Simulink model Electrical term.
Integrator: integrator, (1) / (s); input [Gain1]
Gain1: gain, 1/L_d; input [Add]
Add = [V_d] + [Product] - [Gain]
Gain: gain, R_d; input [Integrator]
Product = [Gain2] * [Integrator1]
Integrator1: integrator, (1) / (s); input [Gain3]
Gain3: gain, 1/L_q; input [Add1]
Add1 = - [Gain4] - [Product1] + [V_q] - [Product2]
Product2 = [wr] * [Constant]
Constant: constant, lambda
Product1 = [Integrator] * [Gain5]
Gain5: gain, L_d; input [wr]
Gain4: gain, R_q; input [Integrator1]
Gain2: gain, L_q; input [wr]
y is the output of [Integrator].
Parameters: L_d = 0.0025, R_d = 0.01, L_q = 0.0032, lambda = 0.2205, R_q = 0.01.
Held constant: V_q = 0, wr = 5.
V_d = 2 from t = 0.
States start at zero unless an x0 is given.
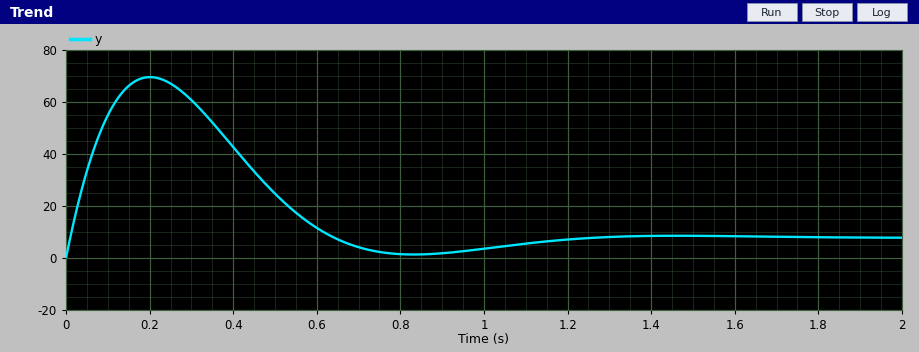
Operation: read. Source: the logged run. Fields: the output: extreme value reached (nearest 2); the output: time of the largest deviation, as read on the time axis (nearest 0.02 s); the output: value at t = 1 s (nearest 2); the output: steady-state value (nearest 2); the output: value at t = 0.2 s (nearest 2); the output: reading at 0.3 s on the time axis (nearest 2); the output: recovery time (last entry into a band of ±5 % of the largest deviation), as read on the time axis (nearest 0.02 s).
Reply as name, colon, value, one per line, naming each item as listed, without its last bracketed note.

the output: extreme value reached: 70
the output: time of the largest deviation, as read on the time axis: 0.20 s
the output: value at t = 1 s: 4
the output: steady-state value: 8
the output: value at t = 0.2 s: 70
the output: reading at 0.3 s on the time axis: 60
the output: recovery time (last entry into a band of ±5 % of the largest deviation), as read on the time axis: 1.04 s
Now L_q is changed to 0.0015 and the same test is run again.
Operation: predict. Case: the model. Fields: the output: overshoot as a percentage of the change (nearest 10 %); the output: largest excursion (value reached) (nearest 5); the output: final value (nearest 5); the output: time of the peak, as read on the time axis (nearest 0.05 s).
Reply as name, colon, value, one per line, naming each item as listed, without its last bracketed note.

the output: overshoot as a percentage of the change: 30 %
the output: largest excursion (value reached): 80
the output: final value: 60
the output: time of the peak, as read on the time axis: 0.25 s
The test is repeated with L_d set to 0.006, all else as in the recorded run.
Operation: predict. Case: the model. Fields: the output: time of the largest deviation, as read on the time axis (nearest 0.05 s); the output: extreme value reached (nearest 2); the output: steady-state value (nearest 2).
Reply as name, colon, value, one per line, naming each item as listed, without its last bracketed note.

the output: time of the largest deviation, as read on the time axis: 0.25 s
the output: extreme value reached: 38
the output: steady-state value: 4
